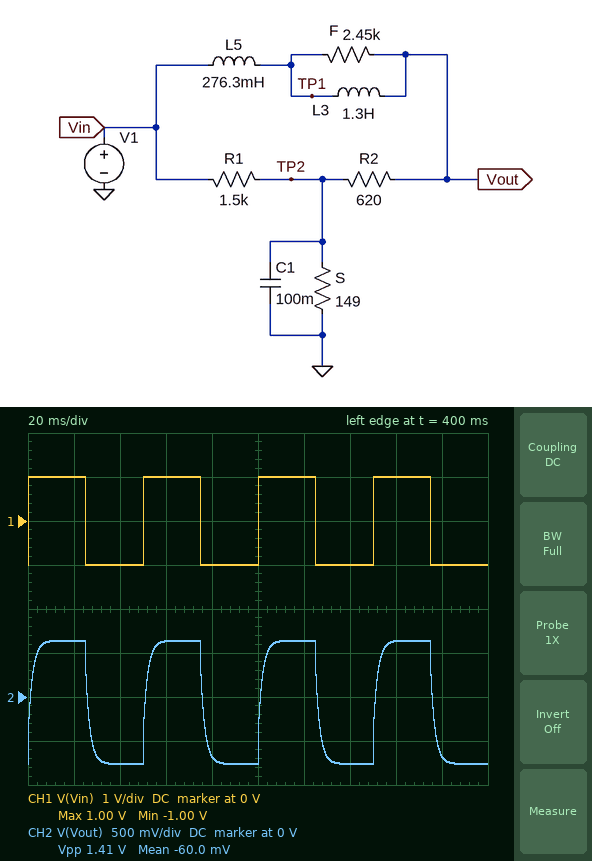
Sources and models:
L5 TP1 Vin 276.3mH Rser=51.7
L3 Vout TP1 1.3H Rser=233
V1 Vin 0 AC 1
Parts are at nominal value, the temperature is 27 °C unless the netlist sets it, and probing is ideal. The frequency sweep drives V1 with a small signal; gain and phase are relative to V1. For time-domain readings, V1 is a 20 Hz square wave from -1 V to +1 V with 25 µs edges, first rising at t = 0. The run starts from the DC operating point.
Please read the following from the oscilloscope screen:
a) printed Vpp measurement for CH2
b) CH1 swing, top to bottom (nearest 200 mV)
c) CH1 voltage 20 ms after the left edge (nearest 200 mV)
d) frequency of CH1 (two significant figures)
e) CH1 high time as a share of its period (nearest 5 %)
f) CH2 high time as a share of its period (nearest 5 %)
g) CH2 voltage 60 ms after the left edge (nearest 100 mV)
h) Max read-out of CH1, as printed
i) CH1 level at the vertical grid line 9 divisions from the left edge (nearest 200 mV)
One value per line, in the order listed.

1.41 V
2.0 V
1.0 V
20 Hz
50 %
50 %
600 mV
1.00 V
-1.0 V
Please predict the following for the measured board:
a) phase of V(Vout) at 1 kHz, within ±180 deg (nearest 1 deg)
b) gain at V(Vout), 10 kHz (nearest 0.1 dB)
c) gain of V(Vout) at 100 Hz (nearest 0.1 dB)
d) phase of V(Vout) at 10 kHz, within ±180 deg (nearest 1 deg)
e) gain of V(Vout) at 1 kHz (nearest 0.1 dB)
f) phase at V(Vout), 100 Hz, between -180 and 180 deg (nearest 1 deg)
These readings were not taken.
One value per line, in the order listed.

-40 deg
-29.1 dB
-6.7 dB
-80 deg
-15.7 dB
-37 deg
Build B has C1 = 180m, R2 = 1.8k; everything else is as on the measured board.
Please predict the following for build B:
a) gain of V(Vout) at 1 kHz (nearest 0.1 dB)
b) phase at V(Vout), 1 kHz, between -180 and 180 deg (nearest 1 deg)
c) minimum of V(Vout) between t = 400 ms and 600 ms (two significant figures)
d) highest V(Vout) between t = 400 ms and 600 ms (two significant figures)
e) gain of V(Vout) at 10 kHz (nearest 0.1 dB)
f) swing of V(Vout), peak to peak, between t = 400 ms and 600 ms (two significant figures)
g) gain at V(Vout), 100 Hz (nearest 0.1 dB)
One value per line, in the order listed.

-8.4 dB
-30 deg
-890 mV
850 mV
-20.0 dB
1.7 V
-2.5 dB
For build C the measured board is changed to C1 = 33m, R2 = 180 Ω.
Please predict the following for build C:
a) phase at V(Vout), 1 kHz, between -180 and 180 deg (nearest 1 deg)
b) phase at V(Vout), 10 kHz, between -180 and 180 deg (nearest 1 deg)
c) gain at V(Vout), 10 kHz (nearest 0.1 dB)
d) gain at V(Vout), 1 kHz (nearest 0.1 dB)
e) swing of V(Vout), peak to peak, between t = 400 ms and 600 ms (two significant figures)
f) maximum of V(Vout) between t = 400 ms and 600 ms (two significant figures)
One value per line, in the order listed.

-44 deg
-81 deg
-39.8 dB
-25.6 dB
820 mV
250 mV
